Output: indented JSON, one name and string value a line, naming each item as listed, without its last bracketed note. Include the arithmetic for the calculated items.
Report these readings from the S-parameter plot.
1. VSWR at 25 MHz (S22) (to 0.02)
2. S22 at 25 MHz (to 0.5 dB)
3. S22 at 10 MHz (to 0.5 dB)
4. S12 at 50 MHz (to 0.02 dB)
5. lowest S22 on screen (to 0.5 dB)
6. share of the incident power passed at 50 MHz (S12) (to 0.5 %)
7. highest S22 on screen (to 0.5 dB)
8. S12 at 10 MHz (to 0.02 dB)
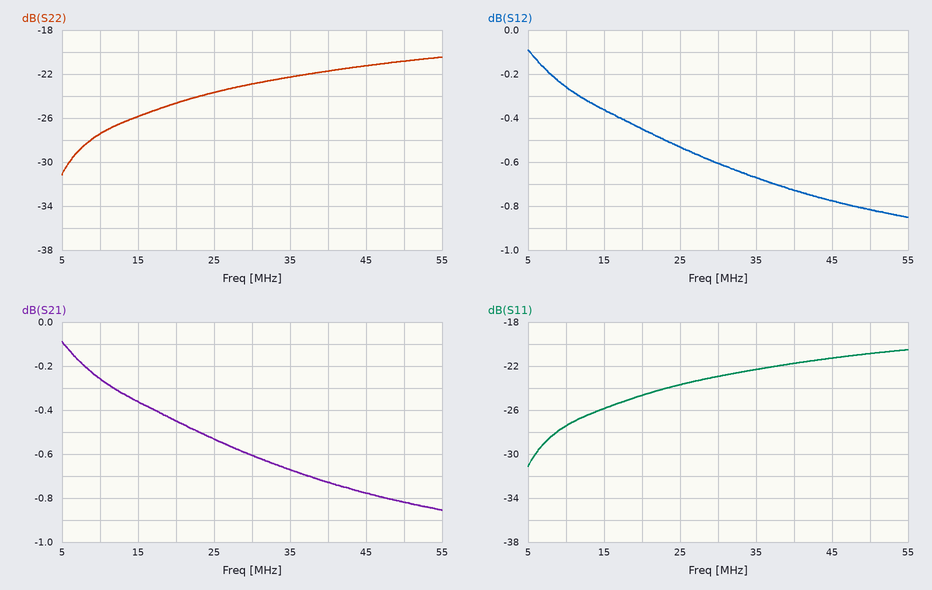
{
  "VSWR at 25 MHz (S22)": "|Γ| = 10^(-23.5/20) = 0.0668; VSWR = (1 + 0.0668)/(1 − 0.0668) ≈ 1.14",
  "S22 at 25 MHz": "-23.5 dB",
  "S22 at 10 MHz": "-27.5 dB",
  "S12 at 50 MHz": "-0.82 dB",
  "lowest S22 on screen": "-31.0 dB",
  "share of the incident power passed at 50 MHz (S12)": "10^(-0.82/10) ≈ 82.8 %, so 83.0 % to the nearest 0.5 %",
  "highest S22 on screen": "-20.5 dB",
  "S12 at 10 MHz": "-0.26 dB"
}
